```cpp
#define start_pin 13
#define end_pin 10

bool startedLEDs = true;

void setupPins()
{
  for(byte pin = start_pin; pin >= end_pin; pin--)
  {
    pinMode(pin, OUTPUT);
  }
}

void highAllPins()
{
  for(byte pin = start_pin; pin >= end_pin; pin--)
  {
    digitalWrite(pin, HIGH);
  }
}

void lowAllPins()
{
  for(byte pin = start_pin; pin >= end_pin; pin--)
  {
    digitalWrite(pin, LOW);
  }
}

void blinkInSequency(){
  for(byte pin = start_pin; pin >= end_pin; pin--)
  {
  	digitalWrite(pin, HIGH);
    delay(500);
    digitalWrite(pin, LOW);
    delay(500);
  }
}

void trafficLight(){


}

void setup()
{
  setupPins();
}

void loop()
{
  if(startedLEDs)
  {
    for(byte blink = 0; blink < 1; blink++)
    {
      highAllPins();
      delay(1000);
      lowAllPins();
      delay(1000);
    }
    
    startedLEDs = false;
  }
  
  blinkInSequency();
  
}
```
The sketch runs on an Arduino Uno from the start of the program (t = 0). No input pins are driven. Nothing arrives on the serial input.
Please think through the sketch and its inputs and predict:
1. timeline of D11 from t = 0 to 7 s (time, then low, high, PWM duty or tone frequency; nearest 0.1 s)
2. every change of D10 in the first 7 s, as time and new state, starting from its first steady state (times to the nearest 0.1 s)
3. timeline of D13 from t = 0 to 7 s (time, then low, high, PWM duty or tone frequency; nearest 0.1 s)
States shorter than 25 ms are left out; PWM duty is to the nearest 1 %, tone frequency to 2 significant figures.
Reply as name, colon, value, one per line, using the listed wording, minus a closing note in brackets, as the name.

timeline of D11 from t = 0 to 7 s: 0 s high; 1 s low; 4 s high; 4.5 s low
every change of D10 in the first 7 s, as time and new state, starting from its first steady state: 0 s high; 1 s low; 5 s high; 5.5 s low
timeline of D13 from t = 0 to 7 s: 0 s high; 1 s low; 2 s high; 2.5 s low; 6 s high; 6.5 s low
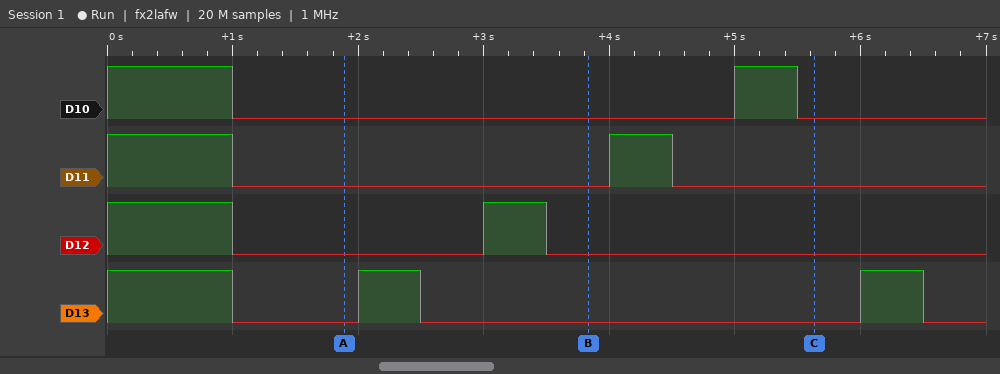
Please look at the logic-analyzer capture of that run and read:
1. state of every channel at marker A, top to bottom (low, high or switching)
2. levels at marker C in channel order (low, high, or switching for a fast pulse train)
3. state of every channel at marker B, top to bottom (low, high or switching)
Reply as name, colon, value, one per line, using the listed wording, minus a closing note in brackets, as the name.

state of every channel at marker A, top to bottom: D10 low, D11 low, D12 low, D13 low
levels at marker C in channel order: D10 low, D11 low, D12 low, D13 low
state of every channel at marker B, top to bottom: D10 low, D11 low, D12 low, D13 low
